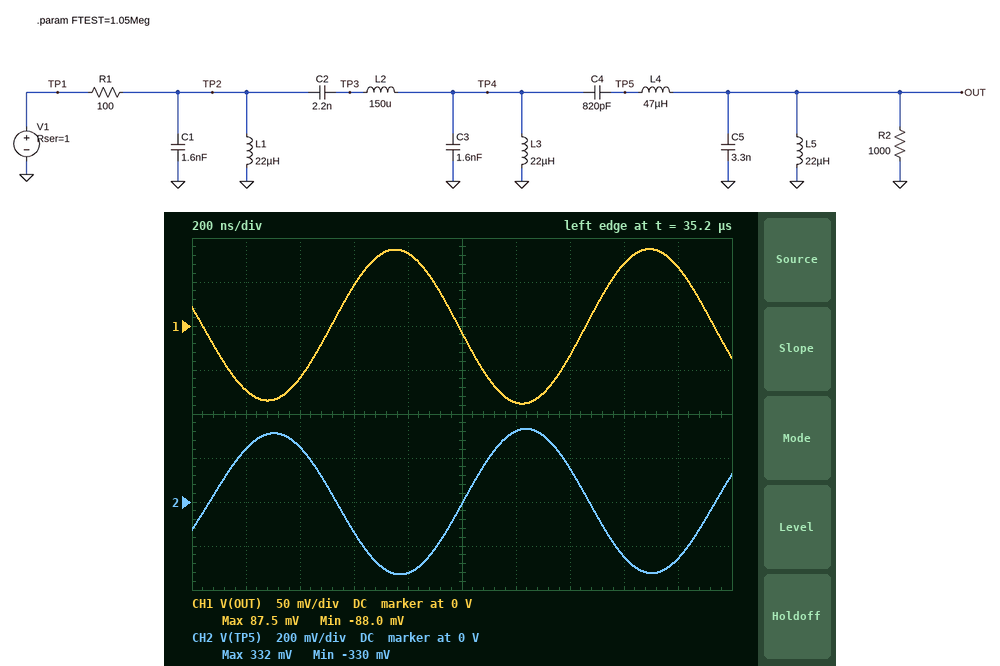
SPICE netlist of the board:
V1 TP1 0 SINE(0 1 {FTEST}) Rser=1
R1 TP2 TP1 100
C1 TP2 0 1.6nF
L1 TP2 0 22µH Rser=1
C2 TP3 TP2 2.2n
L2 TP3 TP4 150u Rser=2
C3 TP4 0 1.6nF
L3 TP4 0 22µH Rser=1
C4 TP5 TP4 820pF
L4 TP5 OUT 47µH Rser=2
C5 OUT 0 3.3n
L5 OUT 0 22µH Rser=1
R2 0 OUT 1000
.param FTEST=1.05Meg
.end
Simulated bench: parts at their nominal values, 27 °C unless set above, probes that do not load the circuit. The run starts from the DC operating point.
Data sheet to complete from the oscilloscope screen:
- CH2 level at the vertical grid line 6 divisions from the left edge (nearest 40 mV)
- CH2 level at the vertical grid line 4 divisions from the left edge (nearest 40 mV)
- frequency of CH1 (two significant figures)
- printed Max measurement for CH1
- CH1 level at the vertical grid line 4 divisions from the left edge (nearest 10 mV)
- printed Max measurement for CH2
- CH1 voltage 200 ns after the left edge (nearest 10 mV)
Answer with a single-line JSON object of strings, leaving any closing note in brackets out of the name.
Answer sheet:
{"CH2 level at the vertical grid line 6 divisions from the left edge": "320 mV", "CH2 level at the vertical grid line 4 divisions from the left edge": "-320 mV", "frequency of CH1": "1.1 MHz", "printed Max measurement for CH1": "87.5 mV", "CH1 level at the vertical grid line 4 divisions from the left edge": "80 mV", "printed Max measurement for CH2": "332 mV", "CH1 voltage 200 ns after the left edge": "-70 mV"}
